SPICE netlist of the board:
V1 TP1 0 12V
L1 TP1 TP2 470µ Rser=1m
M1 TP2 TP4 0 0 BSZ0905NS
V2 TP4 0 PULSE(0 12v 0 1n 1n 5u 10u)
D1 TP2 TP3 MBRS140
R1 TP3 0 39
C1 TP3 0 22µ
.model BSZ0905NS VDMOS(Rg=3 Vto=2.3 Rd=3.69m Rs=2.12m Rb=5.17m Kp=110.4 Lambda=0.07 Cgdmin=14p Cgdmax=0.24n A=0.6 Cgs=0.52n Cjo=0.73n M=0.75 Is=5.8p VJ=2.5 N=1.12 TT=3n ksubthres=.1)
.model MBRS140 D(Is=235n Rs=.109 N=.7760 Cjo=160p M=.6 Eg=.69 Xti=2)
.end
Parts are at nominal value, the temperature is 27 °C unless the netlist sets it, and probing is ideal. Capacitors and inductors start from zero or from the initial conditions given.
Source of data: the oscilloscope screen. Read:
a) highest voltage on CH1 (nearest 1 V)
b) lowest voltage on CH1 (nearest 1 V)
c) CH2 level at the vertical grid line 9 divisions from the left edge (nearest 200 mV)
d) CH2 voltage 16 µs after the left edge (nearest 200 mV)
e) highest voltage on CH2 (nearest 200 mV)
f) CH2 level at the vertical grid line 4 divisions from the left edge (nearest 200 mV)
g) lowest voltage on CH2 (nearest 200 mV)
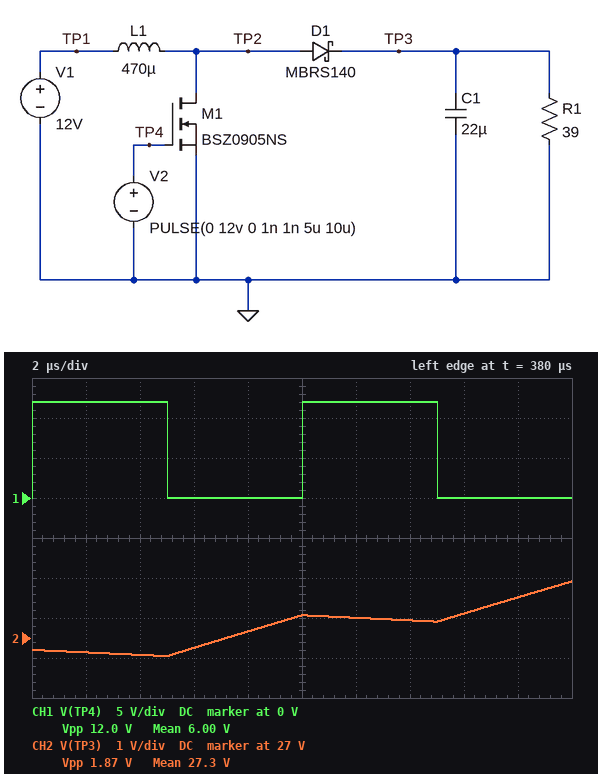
12 V
0 V
28.0 V
27.6 V
28.4 V
27.2 V
26.6 V
